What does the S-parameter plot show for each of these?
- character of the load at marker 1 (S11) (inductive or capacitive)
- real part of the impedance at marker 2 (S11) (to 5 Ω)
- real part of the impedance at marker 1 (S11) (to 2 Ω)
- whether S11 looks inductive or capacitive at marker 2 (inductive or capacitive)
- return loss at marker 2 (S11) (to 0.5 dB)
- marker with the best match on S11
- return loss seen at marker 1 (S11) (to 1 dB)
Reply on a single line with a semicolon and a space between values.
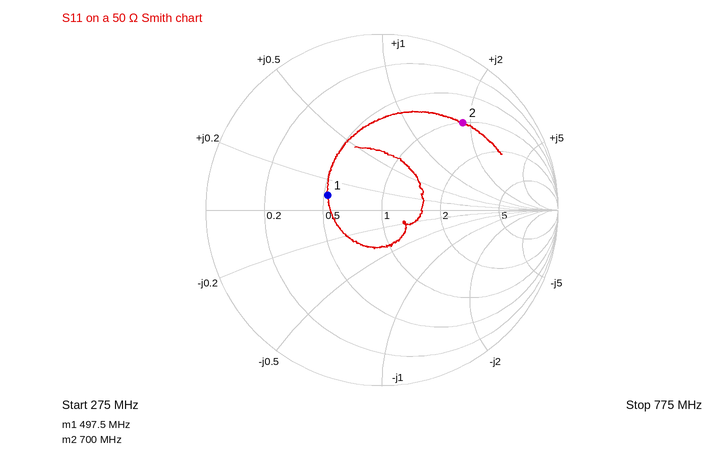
inductive; 50 Ω; 26 Ω; inductive; 3.5 dB; marker 1; 10 dB
